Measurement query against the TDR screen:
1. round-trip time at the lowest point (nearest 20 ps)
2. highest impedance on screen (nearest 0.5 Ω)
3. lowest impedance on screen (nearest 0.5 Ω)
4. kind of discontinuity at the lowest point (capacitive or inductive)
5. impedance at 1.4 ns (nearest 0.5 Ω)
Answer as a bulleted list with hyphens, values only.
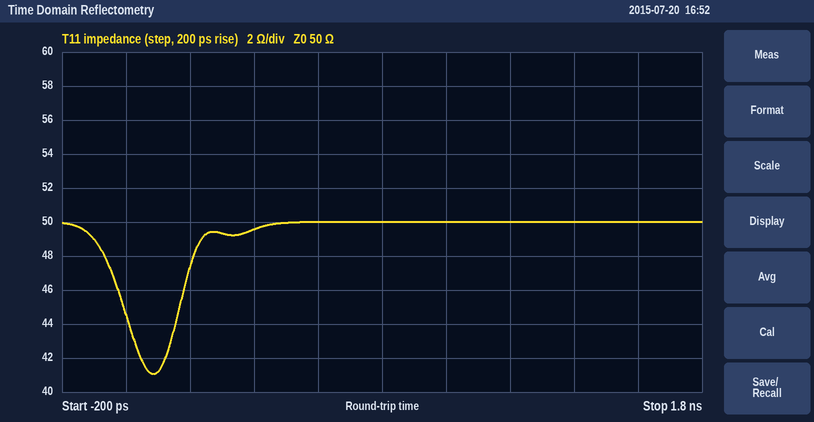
- 80 ps
- 50.0 Ω
- 41.0 Ω
- capacitive
- 50.0 Ω
